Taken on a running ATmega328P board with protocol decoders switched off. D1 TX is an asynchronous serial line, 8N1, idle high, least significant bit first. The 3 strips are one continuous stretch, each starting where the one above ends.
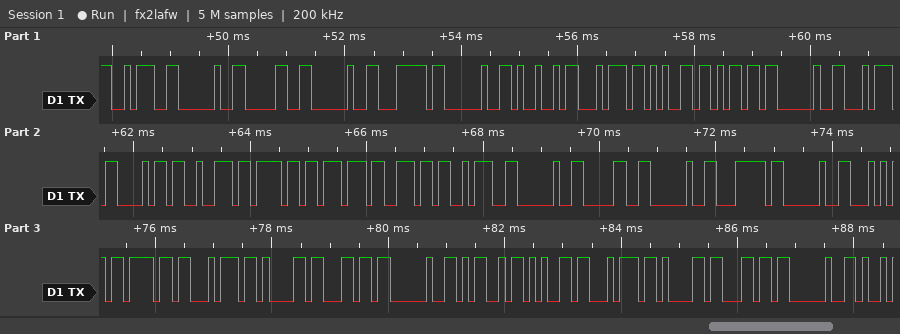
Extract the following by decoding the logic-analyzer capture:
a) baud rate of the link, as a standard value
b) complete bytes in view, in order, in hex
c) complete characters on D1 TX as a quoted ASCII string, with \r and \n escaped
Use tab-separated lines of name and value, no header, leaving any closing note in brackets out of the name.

baud rate of the link, as a standard value	9600 baud
complete bytes in view, in order, in hex	3A 20 30 20 7C 20 49 74 65 6D 20 74 68 72 6F 77 6E 3A 20 30 20 7C 20 54 6F 74 61 6C 20 4D 65 74 61 6C 20
complete characters on D1 TX as a quoted ASCII string, with \r and \n escaped	": 0 | Item thrown: 0 | Total Metal "
